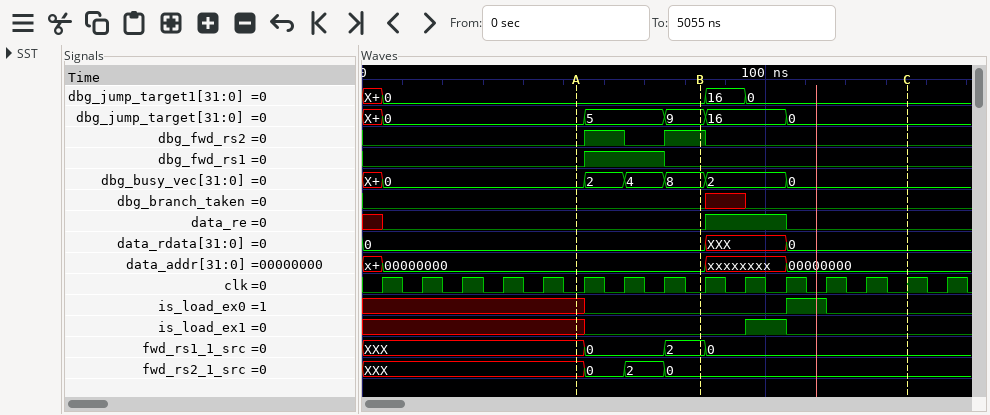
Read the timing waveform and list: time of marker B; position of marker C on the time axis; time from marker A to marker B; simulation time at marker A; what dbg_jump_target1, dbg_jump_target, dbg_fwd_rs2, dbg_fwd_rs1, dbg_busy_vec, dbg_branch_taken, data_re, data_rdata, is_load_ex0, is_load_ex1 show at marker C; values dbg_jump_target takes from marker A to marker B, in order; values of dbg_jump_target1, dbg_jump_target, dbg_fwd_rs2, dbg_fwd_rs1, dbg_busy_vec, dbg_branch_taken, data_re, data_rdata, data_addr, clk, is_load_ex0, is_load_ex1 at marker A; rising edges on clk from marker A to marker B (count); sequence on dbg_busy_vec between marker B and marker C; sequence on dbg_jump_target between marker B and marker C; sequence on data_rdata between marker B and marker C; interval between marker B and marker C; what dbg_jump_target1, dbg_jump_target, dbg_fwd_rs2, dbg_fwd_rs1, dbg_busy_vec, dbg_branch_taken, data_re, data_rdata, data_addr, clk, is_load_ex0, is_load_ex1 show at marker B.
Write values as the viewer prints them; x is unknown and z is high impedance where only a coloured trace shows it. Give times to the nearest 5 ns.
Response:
85 ns
135 ns
30 ns
55 ns
dbg_jump_target1=0, dbg_jump_target=0, dbg_fwd_rs2=0, dbg_fwd_rs1=0, dbg_busy_vec=0, dbg_branch_taken=0, data_re=0, data_rdata=0, is_load_ex0=0, is_load_ex1=0
0, 5, 9
dbg_jump_target1=0, dbg_jump_target=0, dbg_fwd_rs2=0, dbg_fwd_rs1=0, dbg_busy_vec=0, dbg_branch_taken=0, data_re=0, data_rdata=0, data_addr=00000000, clk=0, is_load_ex0=x, is_load_ex1=x
3
8, 2, 0
9, 16, 0
0, XXX, 0
50 ns
dbg_jump_target1=0, dbg_jump_target=9, dbg_fwd_rs2=1, dbg_fwd_rs1=0, dbg_busy_vec=8, dbg_branch_taken=0, data_re=0, data_rdata=0, data_addr=00000000, clk=0, is_load_ex0=0, is_load_ex1=0
